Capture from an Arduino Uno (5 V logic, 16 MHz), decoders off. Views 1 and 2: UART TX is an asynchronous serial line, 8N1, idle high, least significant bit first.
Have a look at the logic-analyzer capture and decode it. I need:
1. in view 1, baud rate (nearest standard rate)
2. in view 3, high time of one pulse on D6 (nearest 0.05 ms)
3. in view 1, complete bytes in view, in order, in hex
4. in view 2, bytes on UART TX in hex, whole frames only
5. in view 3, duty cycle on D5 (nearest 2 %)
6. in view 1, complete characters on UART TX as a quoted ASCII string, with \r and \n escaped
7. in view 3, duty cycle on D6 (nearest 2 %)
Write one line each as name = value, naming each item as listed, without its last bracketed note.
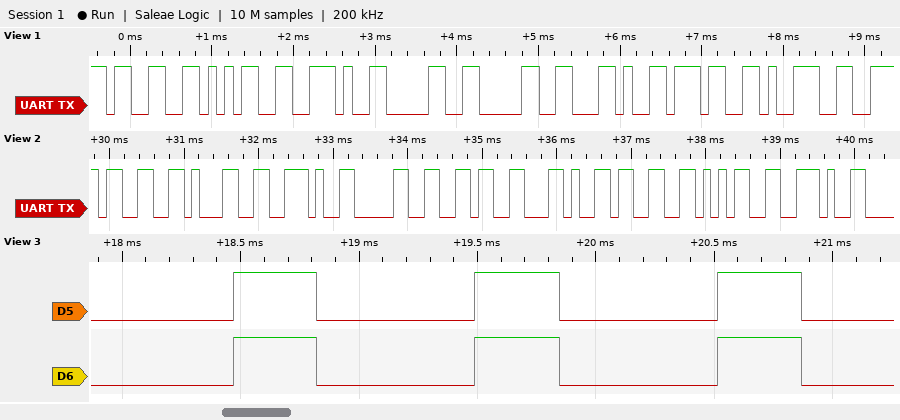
in view 1, baud rate = 9600 baud
in view 3, high time of one pulse on D6 = 0.35 ms
in view 1, complete bytes in view, in order, in hex = 33 35 2E 30 30 2C 37 39
in view 2, bytes on UART TX in hex, whole frames only = 0x33 0x31 0x2E 0x30 0x36 0x2C 0x33 0x35 0x2E
in view 3, duty cycle on D5 = 34 %
in view 1, complete characters on UART TX as a quoted ASCII string, with \r and \n escaped = "35.00,79"
in view 3, duty cycle on D6 = 34 %
